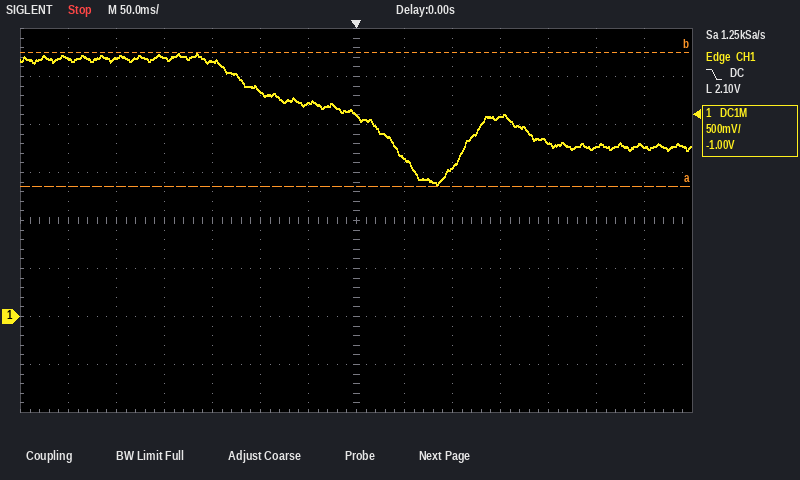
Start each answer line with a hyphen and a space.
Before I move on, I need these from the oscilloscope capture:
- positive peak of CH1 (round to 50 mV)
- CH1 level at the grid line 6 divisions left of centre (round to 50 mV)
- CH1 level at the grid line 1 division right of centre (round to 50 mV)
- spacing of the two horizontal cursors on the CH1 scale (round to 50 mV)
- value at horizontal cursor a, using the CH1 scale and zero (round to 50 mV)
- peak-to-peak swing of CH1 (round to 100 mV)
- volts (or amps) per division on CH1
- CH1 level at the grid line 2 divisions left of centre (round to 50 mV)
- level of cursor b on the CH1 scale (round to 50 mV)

- 2.75 V
- 2.70 V
- 1.65 V
- 1.40 V
- 1.35 V
- 1.40 V
- 500 mV
- 2.35 V
- 2.75 V
